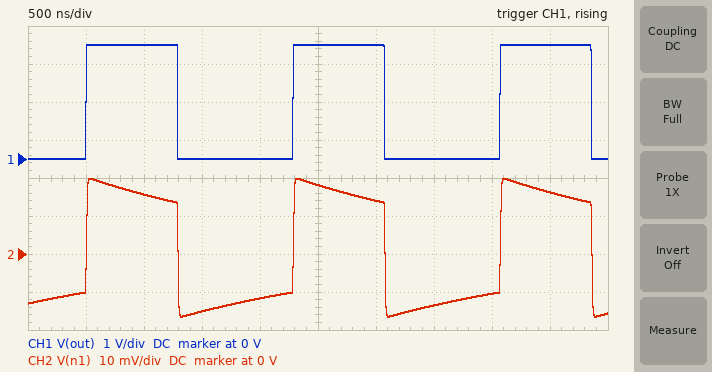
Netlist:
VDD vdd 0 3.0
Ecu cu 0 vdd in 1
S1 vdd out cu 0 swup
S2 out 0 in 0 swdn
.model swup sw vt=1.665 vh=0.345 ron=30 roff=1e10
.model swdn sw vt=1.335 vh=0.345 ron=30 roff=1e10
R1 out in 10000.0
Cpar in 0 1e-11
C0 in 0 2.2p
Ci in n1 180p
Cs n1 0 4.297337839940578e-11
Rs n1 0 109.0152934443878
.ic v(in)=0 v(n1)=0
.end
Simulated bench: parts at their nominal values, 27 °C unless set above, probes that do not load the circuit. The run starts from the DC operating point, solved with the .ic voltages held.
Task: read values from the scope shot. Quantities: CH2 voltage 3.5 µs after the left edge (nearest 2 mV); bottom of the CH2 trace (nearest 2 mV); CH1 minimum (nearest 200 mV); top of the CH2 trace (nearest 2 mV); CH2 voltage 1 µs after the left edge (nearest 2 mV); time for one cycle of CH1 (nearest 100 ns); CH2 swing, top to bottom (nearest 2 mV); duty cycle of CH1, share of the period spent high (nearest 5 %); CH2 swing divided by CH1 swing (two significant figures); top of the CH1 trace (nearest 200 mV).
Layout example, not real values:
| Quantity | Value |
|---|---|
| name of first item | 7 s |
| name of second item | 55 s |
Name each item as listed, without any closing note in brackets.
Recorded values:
| Quantity | Value |
|---|---|
| CH2 voltage 3.5 µs after the left edge | -14 mV |
| bottom of the CH2 trace | -16 mV |
| CH1 minimum | 0 V |
| top of the CH2 trace | 20 mV |
| CH2 voltage 1 µs after the left edge | 16 mV |
| time for one cycle of CH1 | 1.8 µs |
| CH2 swing, top to bottom | 36 mV |
| duty cycle of CH1, share of the period spent high | 45 % |
| CH2 swing divided by CH1 swing | 0.012 |
| top of the CH1 trace | 3.0 V |
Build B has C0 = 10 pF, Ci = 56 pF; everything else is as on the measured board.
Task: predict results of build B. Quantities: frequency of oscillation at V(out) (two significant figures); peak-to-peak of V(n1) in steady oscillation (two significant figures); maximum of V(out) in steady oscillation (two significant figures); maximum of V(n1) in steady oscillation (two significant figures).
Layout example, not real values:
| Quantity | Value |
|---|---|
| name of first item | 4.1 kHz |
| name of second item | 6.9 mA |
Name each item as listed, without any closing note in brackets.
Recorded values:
| Quantity | Value |
|---|---|
| frequency of oscillation at V(out) | 1.4 MHz |
| peak-to-peak of V(n1) in steady oscillation | 28 mV |
| maximum of V(out) in steady oscillation | 3.0 V |
| maximum of V(n1) in steady oscillation | 15 mV |
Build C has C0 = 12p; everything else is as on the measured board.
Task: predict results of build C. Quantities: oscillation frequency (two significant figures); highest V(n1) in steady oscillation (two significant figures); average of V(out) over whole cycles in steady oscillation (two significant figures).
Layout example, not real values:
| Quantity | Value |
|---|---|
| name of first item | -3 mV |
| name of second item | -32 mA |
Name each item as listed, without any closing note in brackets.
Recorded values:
| Quantity | Value |
|---|---|
| oscillation frequency | 530 kHz |
| highest V(n1) in steady oscillation | 19 mV |
| average of V(out) over whole cycles in steady oscillation | 1.3 V |
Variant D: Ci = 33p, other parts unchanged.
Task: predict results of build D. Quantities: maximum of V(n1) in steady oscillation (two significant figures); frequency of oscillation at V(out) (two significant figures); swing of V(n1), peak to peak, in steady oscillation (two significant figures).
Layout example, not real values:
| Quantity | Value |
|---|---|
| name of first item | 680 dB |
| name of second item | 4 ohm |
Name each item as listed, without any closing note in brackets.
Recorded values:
| Quantity | Value |
|---|---|
| maximum of V(n1) in steady oscillation | 15 mV |
| frequency of oscillation at V(out) | 2.4 MHz |
| swing of V(n1), peak to peak, in steady oscillation | 27 mV |
